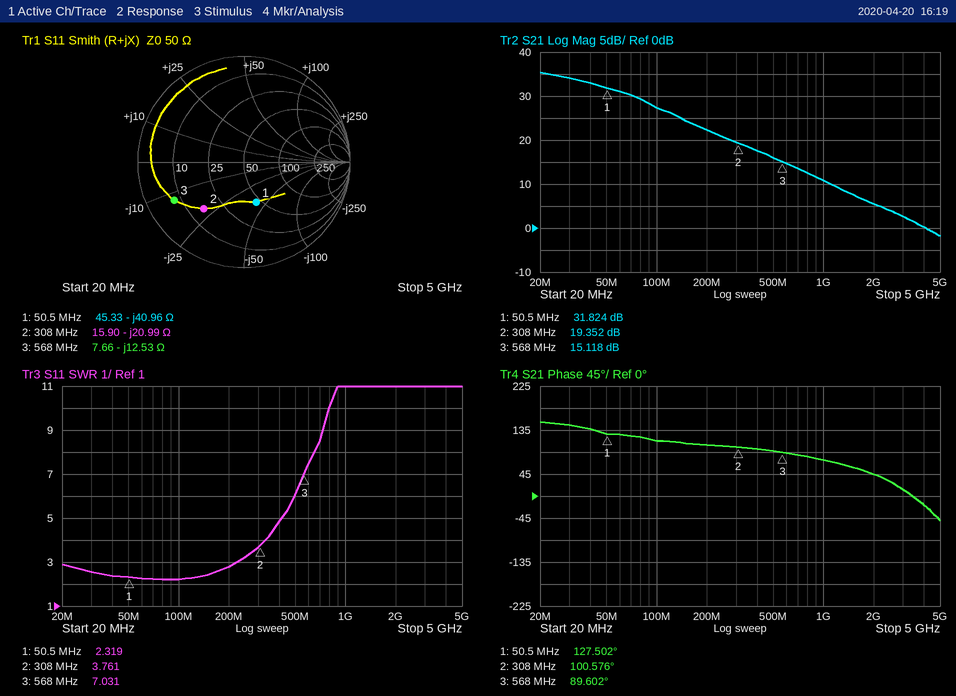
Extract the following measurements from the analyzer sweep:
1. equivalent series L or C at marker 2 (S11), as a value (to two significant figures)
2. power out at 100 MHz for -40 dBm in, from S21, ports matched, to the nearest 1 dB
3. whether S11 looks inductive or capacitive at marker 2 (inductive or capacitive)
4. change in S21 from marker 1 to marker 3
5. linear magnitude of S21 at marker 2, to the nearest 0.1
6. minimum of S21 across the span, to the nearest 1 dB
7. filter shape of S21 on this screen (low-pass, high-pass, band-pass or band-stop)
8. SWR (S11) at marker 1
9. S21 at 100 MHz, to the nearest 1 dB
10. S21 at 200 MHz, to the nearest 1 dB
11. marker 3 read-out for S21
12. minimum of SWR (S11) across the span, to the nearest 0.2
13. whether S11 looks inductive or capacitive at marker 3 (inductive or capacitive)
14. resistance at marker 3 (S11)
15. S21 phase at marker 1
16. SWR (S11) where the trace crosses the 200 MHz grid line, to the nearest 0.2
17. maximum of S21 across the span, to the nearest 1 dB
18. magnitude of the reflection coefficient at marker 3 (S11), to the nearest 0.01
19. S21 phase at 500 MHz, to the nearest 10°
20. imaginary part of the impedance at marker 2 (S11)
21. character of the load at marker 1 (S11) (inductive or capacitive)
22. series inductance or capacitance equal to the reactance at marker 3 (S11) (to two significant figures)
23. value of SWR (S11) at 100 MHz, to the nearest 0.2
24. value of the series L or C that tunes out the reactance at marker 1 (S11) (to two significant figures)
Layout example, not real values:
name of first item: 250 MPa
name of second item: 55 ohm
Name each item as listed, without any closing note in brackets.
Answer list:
equivalent series L or C at marker 2 (S11), as a value: 25 pF
power out at 100 MHz for -40 dBm in, from S21, ports matched, to the nearest 1 dB: -13 dBm
whether S11 looks inductive or capacitive at marker 2: capacitive
change in S21 from marker 1 to marker 3: -16.706 dB
linear magnitude of S21 at marker 2, to the nearest 0.1: 9.3
minimum of S21 across the span, to the nearest 1 dB: -2 dB
filter shape of S21 on this screen: low-pass
SWR (S11) at marker 1: 2.319
S21 at 100 MHz, to the nearest 1 dB: 27 dB
S21 at 200 MHz, to the nearest 1 dB: 22 dB
marker 3 read-out for S21: 15.118 dB
minimum of SWR (S11) across the span, to the nearest 0.2: 2.2
whether S11 looks inductive or capacitive at marker 3: capacitive
resistance at marker 3: 7.66 Ω
S21 phase at marker 1: 127.502°
SWR (S11) where the trace crosses the 200 MHz grid line, to the nearest 0.2: 2.8
maximum of S21 across the span, to the nearest 1 dB: 35 dB
magnitude of the reflection coefficient at marker 3 (S11), to the nearest 0.01: 0.75
S21 phase at 500 MHz, to the nearest 10°: 90°
imaginary part of the impedance at marker 2: -20.99 Ω
character of the load at marker 1 (S11): capacitive
series inductance or capacitance equal to the reactance at marker 3 (S11): 22 pF
value of SWR (S11) at 100 MHz, to the nearest 0.2: 2.2
value of the series L or C that tunes out the reactance at marker 1 (S11): 130 nH
